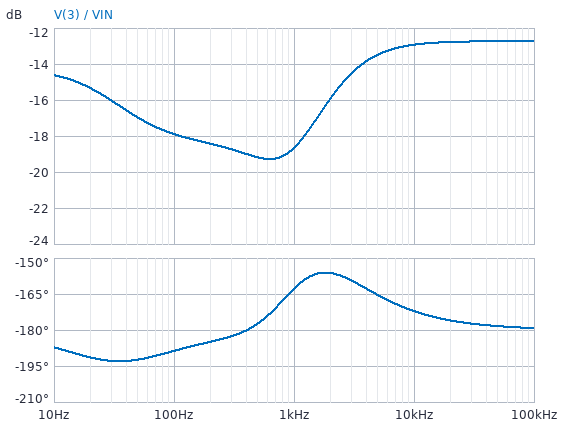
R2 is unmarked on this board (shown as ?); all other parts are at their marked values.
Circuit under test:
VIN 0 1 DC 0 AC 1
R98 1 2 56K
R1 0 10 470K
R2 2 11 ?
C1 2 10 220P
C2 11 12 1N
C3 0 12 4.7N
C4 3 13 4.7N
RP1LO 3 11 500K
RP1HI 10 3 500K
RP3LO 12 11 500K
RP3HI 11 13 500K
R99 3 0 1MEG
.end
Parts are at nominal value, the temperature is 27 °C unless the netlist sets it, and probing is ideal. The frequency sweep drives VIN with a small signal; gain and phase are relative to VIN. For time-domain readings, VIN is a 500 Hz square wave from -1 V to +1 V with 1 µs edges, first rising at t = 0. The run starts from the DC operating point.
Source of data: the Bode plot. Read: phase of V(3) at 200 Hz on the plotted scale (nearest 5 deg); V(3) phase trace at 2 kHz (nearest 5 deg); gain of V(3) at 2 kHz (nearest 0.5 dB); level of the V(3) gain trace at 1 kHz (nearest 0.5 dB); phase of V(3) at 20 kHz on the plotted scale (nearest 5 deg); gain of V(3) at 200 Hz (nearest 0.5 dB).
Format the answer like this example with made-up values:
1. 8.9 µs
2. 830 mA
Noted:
1. -185 deg
2. -155 deg
3. -16.0 dB
4. -18.5 dB
5. -175 deg
6. -18.5 dB
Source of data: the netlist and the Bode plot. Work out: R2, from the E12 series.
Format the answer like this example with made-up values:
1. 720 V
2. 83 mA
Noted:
1. 1.5 MΩ
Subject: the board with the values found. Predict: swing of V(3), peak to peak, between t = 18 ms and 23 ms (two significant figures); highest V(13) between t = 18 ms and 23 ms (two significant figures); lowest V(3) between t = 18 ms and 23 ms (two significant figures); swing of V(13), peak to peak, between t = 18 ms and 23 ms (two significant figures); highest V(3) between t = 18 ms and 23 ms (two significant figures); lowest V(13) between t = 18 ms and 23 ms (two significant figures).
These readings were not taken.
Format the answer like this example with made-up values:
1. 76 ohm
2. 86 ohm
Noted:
1. 670 mV
2. 340 mV
3. -330 mV
4. 670 mV
5. 340 mV
6. -320 mV
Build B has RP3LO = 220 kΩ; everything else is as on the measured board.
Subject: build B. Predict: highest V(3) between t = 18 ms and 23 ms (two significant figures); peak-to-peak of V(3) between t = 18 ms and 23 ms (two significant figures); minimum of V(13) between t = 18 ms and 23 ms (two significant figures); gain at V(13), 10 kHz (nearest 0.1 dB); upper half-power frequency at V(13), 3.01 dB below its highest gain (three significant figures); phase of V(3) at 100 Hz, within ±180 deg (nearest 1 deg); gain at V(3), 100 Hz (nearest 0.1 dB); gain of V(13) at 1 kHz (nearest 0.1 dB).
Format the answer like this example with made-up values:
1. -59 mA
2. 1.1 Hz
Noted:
1. 370 mV
2. 730 mV
3. -360 mV
4. -12.9 dB
5. 28.5 Hz
6. 160 deg
7. -19.5 dB
8. -18.9 dB
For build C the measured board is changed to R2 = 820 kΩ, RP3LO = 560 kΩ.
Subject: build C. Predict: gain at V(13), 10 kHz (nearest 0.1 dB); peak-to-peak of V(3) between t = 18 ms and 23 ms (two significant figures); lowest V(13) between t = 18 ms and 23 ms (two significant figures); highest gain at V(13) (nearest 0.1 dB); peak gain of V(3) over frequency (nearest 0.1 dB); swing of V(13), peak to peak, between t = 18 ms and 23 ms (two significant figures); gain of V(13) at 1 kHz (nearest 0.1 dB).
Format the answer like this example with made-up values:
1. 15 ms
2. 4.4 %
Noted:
1. -13.2 dB
2. 500 mV
3. -230 mV
4. -5.5 dB
5. -11.6 dB
6. 480 mV
7. -18.0 dB
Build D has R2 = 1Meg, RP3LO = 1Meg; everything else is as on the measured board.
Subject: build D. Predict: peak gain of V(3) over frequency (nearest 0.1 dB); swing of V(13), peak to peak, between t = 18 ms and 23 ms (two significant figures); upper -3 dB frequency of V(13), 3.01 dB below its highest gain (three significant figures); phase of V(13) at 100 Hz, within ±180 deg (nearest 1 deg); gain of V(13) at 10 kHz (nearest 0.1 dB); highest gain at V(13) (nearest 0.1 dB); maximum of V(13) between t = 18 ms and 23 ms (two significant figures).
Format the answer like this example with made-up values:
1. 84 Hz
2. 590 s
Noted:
1. -12.4 dB
2. 500 mV
3. 29.8 Hz
4. 157 deg
5. -13.1 dB
6. -6.3 dB
7. 260 mV
